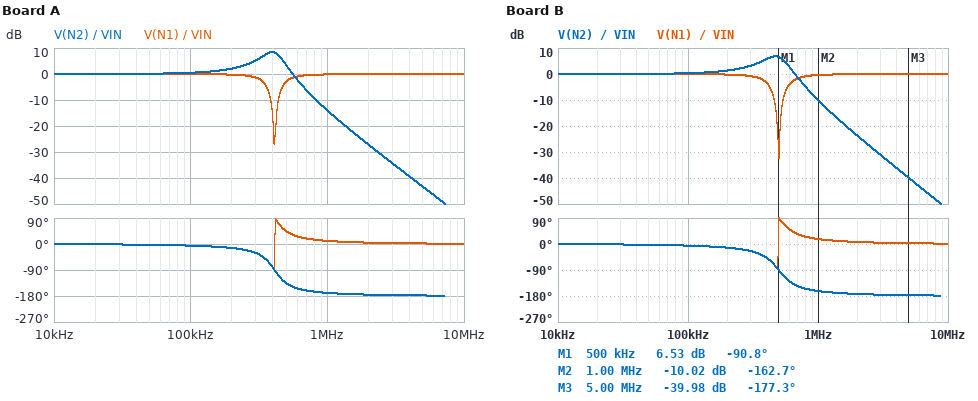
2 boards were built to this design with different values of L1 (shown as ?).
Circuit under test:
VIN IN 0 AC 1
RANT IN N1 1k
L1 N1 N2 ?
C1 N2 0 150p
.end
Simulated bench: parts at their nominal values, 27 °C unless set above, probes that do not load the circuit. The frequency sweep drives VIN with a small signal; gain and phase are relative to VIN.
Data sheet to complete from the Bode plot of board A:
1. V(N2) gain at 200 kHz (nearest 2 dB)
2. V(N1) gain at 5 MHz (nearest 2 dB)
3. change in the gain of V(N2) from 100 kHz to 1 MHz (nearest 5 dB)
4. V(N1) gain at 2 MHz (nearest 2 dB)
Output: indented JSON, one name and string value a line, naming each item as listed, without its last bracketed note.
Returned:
{
  "V(N2) gain at 200 kHz": "2 dB",
  "V(N1) gain at 5 MHz": "0 dB",
  "change in the gain of V(N2) from 100 kHz to 1 MHz": "-15 dB",
  "V(N1) gain at 2 MHz": "0 dB"
}
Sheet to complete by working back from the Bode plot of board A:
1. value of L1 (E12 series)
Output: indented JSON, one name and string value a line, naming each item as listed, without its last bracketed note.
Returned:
{
  "value of L1": "1 mH"
}
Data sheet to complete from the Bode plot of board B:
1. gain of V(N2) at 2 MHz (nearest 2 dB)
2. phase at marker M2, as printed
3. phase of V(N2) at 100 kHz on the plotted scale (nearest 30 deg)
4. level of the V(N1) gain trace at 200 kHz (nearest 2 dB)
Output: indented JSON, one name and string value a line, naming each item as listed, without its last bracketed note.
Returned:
{
  "gain of V(N2) at 2 MHz": "-24 dB",
  "phase at marker M2, as printed": "-162.7 deg",
  "phase of V(N2) at 100 kHz on the plotted scale": "0 deg",
  "level of the V(N1) gain trace at 200 kHz": "0 dB"
}
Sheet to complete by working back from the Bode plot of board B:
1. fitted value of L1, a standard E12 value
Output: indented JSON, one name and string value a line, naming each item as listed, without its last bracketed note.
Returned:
{
  "fitted value of L1, a standard E12 value": "680 µH"
}
